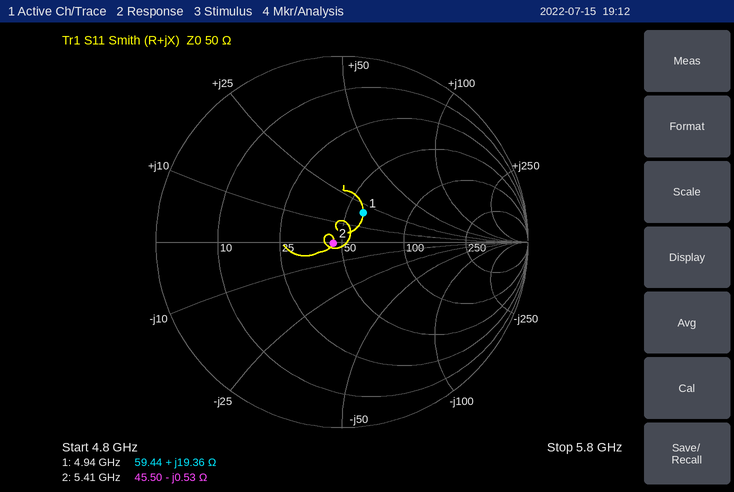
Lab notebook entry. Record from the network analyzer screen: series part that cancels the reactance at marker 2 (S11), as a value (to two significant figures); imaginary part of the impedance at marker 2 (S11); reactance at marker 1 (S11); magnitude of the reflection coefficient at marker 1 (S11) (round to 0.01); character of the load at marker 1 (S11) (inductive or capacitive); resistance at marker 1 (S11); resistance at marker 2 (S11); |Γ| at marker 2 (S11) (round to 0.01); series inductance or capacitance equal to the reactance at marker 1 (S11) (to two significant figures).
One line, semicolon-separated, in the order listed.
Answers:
16 pH; -0.53 Ω; +19.36 Ω; 0.19; inductive; 59.44 Ω; 45.50 Ω; 0.05; 620 pH
